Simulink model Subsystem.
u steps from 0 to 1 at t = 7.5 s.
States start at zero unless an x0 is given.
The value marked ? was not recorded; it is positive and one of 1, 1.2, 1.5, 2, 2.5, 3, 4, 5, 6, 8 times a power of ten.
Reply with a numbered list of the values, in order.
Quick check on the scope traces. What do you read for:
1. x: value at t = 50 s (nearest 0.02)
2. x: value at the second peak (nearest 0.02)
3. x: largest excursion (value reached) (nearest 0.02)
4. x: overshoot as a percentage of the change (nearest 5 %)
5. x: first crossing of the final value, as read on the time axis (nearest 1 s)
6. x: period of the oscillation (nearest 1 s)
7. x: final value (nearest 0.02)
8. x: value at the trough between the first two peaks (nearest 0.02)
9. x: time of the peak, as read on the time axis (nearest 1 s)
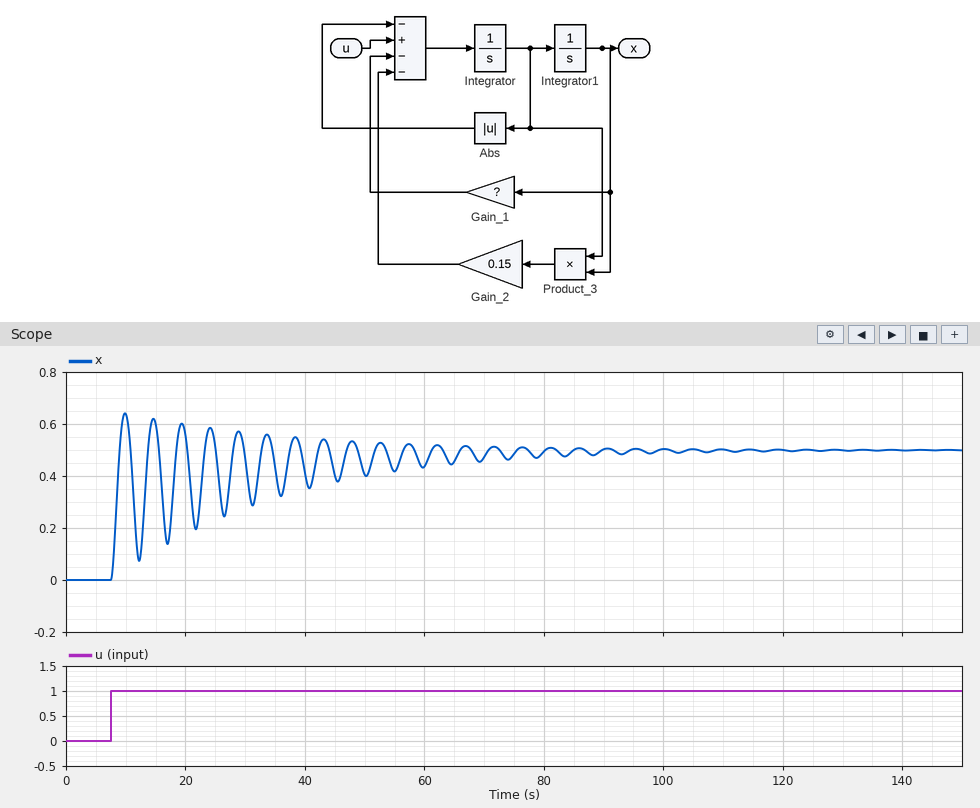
1. 0.40
2. 0.62
3. 0.64
4. 30 %
5. 9 s
6. 5 s
7. 0.50
8. 0.08
9. 10 s
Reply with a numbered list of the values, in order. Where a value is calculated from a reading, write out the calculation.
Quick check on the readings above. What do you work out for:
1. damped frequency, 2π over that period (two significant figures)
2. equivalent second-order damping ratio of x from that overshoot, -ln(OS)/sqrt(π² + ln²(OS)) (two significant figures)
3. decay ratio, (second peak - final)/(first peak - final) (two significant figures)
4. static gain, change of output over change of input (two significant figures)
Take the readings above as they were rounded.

1. 2π / 5 = 1.3 rad/s
2. ln(0.3) = -1.204; 1.204 / sqrt(9.870 + 1.450) = 0.36
3. (0.62 - 0.5) / (0.64 - 0.5) = 0.86
4. (0.5 - 0) / (1 - 0) = 0.50
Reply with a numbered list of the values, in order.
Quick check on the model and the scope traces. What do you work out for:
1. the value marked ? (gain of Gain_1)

1. 2
